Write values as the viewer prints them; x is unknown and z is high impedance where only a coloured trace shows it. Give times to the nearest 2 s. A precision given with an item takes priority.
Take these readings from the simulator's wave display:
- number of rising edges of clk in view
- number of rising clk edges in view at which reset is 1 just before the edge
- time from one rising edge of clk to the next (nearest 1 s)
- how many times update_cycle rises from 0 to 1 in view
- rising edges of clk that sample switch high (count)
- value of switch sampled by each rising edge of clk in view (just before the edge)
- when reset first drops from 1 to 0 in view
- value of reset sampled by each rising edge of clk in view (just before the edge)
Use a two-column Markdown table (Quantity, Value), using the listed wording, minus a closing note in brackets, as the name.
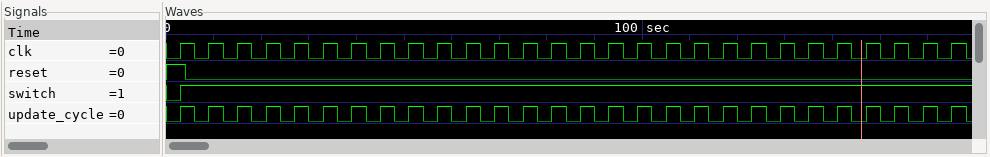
| Quantity | Value |
|---|---|
| number of rising edges of clk in view | 28 |
| number of rising clk edges in view at which reset is 1 just before the edge | 1 |
| time from one rising edge of clk to the next | 6 s |
| how many times update_cycle rises from 0 to 1 in view | 28 |
| rising edges of clk that sample switch high | 27 |
| value of switch sampled by each rising edge of clk in view | 0 1 1 1 1 1 1 1 1 1 1 1 1 1 1 1 1 1 1 1 1 1 1 1 1 1 1 1 |
| when reset first drops from 1 to 0 in view | 4 s |
| value of reset sampled by each rising edge of clk in view | 1 0 0 0 0 0 0 0 0 0 0 0 0 0 0 0 0 0 0 0 0 0 0 0 0 0 0 0 |
